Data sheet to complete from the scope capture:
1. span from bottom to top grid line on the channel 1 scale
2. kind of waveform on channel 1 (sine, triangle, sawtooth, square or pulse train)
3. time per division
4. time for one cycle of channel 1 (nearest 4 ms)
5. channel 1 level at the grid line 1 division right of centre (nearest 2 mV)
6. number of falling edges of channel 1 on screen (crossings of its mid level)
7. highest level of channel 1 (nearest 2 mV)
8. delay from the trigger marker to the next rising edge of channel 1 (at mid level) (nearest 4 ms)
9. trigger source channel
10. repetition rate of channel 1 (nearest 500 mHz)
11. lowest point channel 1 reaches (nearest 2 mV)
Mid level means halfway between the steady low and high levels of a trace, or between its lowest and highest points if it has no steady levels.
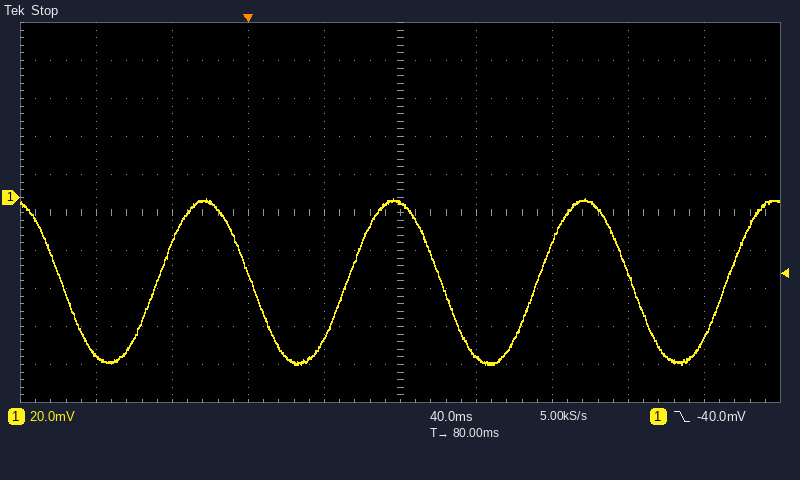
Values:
200 mV
sine
40 ms
100 ms
-84 mV
4
0 mV
52 ms
channel 1
10.0 Hz
-88 mV
